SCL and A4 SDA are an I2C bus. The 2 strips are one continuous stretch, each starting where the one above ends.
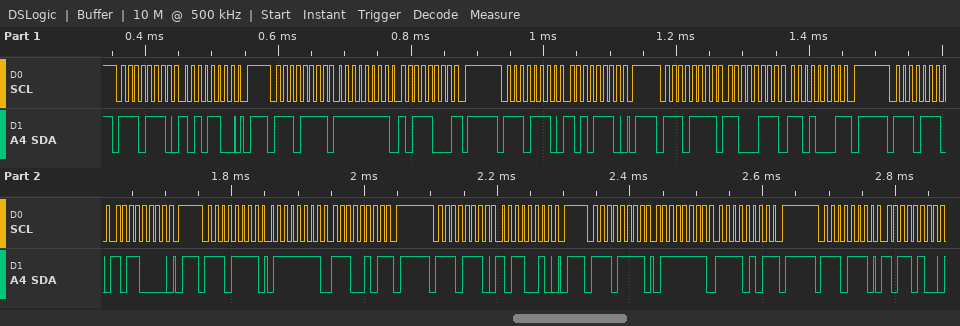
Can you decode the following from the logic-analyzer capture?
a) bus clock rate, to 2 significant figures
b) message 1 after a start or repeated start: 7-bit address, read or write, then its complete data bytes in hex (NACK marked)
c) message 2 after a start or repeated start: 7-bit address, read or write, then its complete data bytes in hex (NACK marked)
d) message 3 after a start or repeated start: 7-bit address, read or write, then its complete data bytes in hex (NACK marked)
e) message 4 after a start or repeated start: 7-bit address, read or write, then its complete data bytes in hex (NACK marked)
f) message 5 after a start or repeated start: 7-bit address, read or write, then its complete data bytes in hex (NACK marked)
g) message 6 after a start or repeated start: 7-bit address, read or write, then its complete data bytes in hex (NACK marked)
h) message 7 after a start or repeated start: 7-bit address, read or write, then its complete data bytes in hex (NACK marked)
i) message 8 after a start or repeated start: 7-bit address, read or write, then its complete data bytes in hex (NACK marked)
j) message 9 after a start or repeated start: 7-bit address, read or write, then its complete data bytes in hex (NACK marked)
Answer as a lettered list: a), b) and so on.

a) 100 kHz
b) 0x77 write: AC
c) 0x77 read: FF B8 NACK
d) 0x77 write: AE
e) 0x77 read: C7 D1 NACK
f) 0x77 write: B0
g) 0x77 read: 7F E5 NACK
h) 0x77 write: B2
i) 0x77 read: 7F F5 NACK
j) 0x77 write: B4
